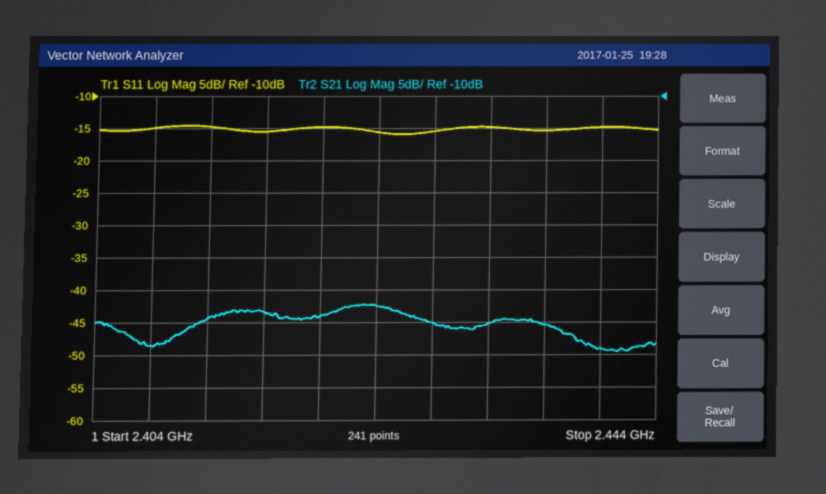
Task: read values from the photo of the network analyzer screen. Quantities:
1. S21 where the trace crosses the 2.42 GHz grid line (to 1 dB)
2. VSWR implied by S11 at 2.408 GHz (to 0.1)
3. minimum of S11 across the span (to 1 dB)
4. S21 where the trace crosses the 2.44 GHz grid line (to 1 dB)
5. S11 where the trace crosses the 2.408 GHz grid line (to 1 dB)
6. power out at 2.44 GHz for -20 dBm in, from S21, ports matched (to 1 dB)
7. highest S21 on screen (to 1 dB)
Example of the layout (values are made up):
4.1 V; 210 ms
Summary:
-44 dB; 1.4; -16 dB; -49 dB; -15 dB; -69 dBm; -42 dB
